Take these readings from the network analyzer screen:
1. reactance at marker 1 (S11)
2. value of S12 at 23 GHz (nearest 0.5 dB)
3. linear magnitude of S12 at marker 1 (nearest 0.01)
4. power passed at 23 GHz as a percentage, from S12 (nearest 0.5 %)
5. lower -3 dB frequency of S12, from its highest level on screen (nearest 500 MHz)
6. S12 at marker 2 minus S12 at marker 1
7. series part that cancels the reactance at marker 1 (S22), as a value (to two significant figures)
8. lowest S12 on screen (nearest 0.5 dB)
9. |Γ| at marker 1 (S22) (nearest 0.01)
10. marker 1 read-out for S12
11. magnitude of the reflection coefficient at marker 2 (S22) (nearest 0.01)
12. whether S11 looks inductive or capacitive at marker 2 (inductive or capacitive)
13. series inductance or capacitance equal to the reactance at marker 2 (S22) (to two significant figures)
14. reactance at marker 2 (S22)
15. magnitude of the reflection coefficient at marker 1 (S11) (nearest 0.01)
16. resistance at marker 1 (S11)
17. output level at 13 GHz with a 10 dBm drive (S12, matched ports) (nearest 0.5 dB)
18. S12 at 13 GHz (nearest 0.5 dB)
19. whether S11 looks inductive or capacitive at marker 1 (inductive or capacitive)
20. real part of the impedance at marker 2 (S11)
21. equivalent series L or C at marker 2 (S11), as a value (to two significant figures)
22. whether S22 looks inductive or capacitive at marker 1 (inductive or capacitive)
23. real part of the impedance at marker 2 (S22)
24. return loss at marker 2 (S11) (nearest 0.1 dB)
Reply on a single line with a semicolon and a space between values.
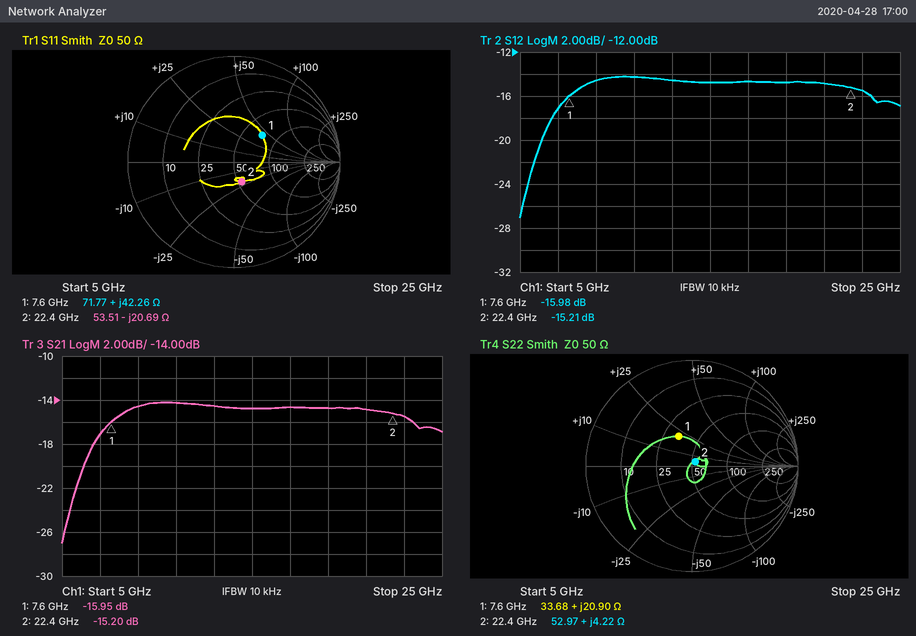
+42.26 Ω; -15.5 dB; 0.16; 3.0 %; 7.0 GHz; 0.77 dB; 1.0 pF; -27.0 dB; 0.31; -15.98 dB; 0.05; capacitive; 30 pH; +4.22 Ω; 0.37; 71.77 Ω; -4.5 dBm; -14.5 dB; inductive; 53.51 Ω; 340 fF; inductive; 52.97 Ω; 14.0 dB
